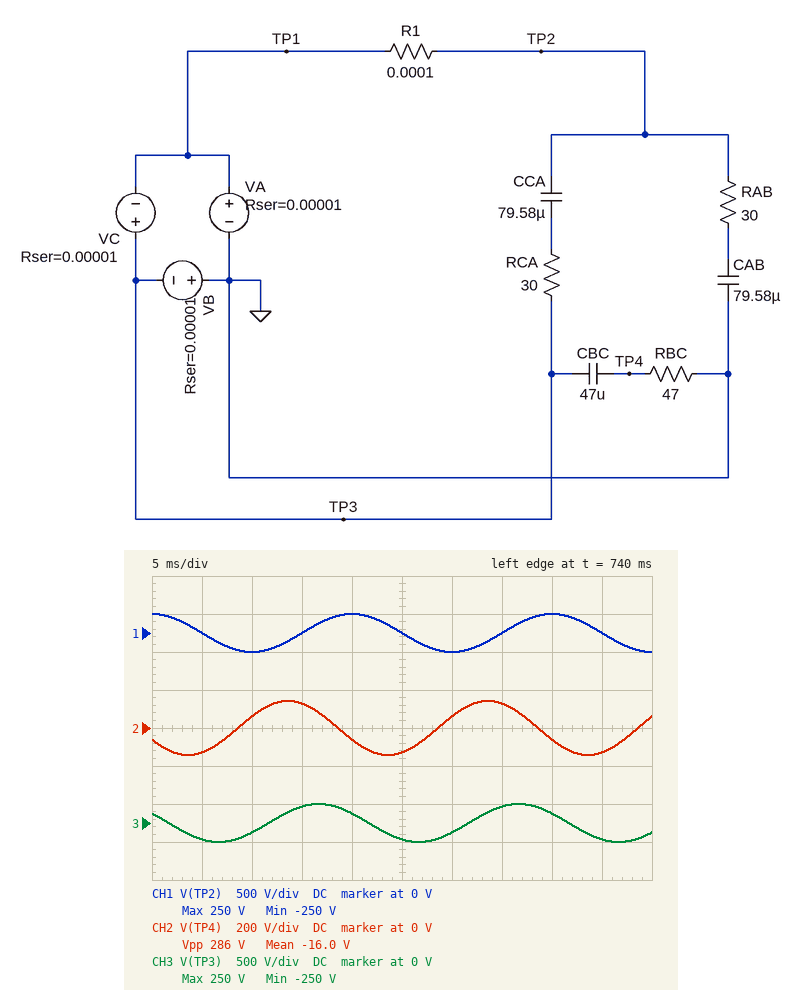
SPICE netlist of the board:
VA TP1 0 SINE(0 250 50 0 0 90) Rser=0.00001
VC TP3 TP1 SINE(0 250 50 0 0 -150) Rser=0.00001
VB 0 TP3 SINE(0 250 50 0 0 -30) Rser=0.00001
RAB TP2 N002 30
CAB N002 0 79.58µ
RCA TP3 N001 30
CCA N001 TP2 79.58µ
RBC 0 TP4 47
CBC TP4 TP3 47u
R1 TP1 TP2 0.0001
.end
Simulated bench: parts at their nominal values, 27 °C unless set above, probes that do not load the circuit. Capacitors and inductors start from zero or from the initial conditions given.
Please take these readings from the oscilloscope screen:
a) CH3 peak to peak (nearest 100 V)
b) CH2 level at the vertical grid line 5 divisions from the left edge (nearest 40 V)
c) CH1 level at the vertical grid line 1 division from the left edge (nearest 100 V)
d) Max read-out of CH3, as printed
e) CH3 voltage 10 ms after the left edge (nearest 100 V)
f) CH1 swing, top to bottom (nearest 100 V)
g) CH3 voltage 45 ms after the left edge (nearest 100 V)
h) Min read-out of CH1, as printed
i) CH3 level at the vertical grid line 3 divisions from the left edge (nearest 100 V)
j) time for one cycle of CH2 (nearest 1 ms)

500 V
-120 V
0 V
250 V
-100 V
500 V
-200 V
-250 V
200 V
20 ms
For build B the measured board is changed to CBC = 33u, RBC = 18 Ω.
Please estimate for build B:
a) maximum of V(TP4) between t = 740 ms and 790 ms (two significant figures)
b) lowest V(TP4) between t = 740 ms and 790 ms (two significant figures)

46 V
-46 V
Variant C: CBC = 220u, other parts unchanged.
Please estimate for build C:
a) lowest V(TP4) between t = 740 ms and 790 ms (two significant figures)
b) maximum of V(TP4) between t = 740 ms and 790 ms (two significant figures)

-240 V
240 V
